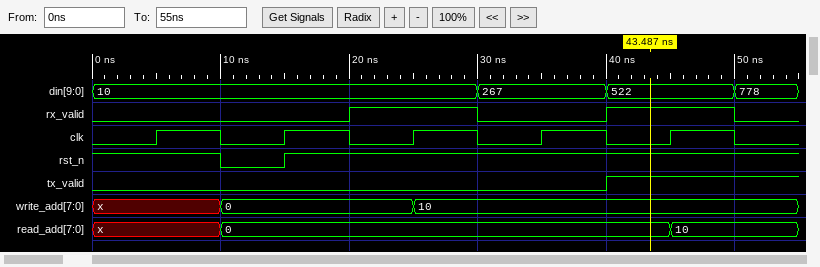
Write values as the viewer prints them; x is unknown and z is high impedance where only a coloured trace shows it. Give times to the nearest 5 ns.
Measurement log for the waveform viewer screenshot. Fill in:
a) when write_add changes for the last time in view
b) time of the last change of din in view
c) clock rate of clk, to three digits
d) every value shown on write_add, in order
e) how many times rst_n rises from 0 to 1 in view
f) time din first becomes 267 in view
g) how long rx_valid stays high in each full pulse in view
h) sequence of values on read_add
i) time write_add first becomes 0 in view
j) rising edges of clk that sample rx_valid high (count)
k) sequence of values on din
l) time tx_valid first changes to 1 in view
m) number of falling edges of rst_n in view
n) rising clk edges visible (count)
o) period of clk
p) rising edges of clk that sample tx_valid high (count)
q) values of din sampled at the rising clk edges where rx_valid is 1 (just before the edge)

25 ns
50 ns
100 MHz
x, 0, 10
1
30 ns
10 ns, 10 ns
x, 0, 10
10 ns
2
10, 267, 522, 778
40 ns
1
5
10 ns
1
10, 522
